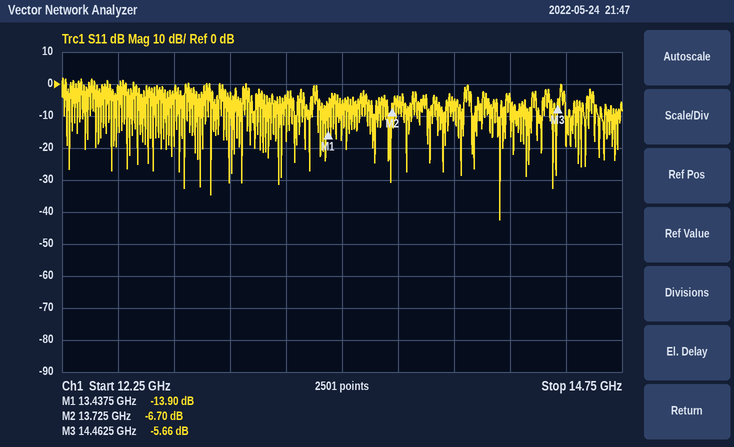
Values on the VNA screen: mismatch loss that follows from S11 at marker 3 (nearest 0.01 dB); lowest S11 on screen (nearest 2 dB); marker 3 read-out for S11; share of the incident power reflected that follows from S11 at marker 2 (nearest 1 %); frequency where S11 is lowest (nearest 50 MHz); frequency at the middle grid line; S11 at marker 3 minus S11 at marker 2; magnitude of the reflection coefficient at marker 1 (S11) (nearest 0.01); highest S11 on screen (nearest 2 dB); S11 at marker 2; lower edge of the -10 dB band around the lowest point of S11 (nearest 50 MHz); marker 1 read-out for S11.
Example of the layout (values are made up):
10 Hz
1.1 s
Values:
1.38 dB
-42 dB
-5.66 dB
21 %
14.20 GHz
13.5 GHz
1.04 dB
0.20
2 dB
-6.70 dB
14.20 GHz
-13.90 dB
